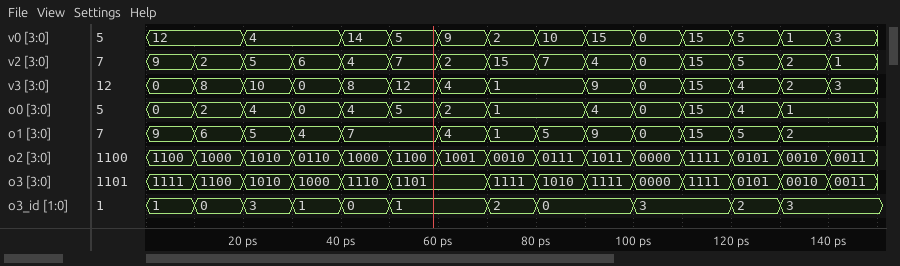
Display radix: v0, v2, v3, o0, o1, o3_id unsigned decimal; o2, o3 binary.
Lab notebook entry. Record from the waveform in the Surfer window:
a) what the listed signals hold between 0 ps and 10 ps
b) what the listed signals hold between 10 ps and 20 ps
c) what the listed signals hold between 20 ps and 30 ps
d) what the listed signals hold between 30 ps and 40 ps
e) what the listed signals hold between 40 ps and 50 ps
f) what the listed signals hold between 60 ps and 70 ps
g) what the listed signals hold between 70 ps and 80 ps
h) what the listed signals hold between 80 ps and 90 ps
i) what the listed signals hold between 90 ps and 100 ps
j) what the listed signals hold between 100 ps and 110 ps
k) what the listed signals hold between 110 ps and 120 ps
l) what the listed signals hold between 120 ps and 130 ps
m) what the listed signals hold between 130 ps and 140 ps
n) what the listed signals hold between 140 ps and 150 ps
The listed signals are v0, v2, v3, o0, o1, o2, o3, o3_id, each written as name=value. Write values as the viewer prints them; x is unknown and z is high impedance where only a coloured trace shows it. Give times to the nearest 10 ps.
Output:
v0=12, v2=9, v3=0, o0=0, o1=9, o2=1100, o3=1111, o3_id=1
v0=12, v2=2, v3=8, o0=2, o1=6, o2=1000, o3=1100, o3_id=0
v0=4, v2=5, v3=10, o0=4, o1=5, o2=1010, o3=1010, o3_id=3
v0=4, v2=6, v3=0, o0=0, o1=4, o2=0110, o3=1000, o3_id=1
v0=14, v2=4, v3=8, o0=4, o1=7, o2=1000, o3=1110, o3_id=0
v0=9, v2=2, v3=4, o0=2, o1=4, o2=1001, o3=1101, o3_id=1
v0=2, v2=15, v3=1, o0=1, o1=1, o2=0010, o3=1111, o3_id=2
v0=10, v2=7, v3=1, o0=1, o1=5, o2=0111, o3=1010, o3_id=0
v0=15, v2=4, v3=9, o0=4, o1=9, o2=1011, o3=1111, o3_id=0
v0=0, v2=0, v3=0, o0=0, o1=0, o2=0000, o3=0000, o3_id=3
v0=15, v2=15, v3=15, o0=15, o1=15, o2=1111, o3=1111, o3_id=3
v0=5, v2=5, v3=4, o0=4, o1=5, o2=0101, o3=0101, o3_id=2
v0=1, v2=2, v3=2, o0=1, o1=2, o2=0010, o3=0010, o3_id=3
v0=3, v2=1, v3=3, o0=1, o1=2, o2=0011, o3=0011, o3_id=3
